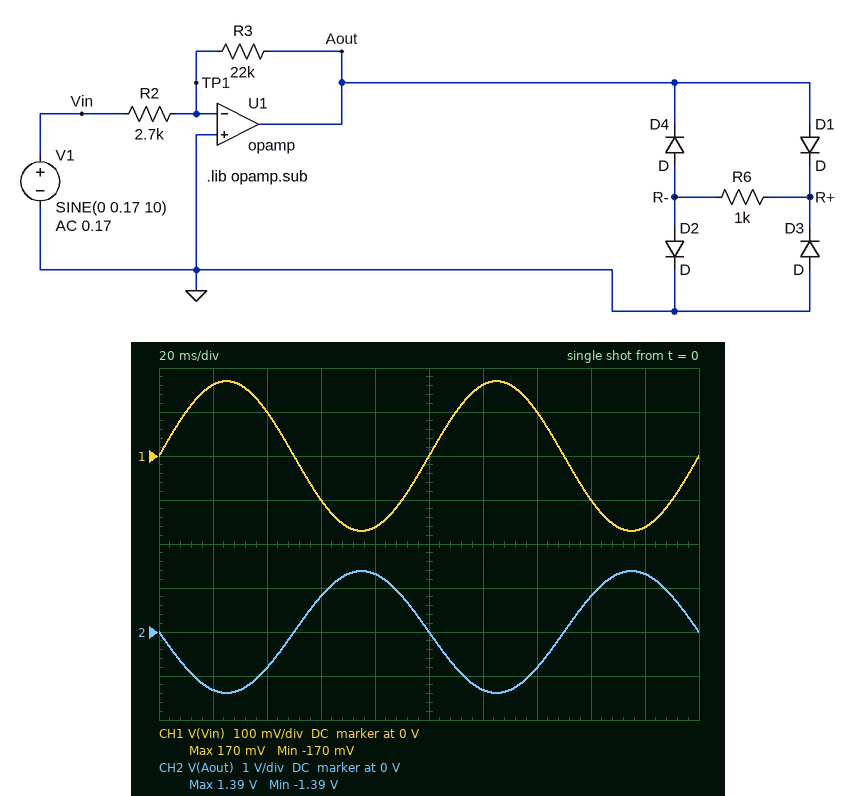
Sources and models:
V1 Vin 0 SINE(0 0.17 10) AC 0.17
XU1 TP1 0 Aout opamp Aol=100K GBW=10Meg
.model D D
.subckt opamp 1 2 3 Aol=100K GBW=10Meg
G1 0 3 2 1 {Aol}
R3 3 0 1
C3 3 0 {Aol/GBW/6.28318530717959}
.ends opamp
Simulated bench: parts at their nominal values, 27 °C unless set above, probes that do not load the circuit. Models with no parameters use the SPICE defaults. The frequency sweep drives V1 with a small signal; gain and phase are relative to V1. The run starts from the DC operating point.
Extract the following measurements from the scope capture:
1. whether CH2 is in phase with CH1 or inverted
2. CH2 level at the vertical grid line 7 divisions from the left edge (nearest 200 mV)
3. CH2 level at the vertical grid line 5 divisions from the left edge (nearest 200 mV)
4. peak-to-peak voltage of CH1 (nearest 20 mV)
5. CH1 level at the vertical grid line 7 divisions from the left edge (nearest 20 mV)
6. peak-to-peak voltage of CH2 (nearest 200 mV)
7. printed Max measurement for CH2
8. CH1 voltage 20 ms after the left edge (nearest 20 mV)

inverted
-800 mV
0 V
340 mV
100 mV
2.8 V
1.39 V
160 mV
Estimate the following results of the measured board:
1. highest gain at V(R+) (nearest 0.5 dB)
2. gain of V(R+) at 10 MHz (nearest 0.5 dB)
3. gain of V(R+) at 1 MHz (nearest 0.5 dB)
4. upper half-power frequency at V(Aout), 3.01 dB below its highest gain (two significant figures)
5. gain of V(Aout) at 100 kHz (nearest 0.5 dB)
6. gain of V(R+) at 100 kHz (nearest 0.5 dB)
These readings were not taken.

12.0 dB
-7.0 dB
9.5 dB
1.1 MHz
18.0 dB
12.0 dB
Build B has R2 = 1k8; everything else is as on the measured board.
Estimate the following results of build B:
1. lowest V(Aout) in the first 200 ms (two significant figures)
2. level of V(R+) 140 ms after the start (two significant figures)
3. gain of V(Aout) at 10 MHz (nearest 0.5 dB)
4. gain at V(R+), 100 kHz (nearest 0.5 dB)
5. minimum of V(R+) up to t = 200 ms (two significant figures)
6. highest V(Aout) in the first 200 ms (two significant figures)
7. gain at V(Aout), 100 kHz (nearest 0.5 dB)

-2.1 V
-580 mV
-0.5 dB
15.5 dB
-650 mV
2.1 V
21.5 dB
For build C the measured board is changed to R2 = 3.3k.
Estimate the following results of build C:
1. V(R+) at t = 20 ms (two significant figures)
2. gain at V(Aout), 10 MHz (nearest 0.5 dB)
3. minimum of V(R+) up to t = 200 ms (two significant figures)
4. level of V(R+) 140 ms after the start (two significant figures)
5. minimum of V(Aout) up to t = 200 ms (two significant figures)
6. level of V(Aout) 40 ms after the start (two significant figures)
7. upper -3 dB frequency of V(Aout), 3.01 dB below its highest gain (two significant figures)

-530 mV
-1.5 dB
-560 mV
-330 mV
-1.1 V
-670 mV
1.3 MHz
